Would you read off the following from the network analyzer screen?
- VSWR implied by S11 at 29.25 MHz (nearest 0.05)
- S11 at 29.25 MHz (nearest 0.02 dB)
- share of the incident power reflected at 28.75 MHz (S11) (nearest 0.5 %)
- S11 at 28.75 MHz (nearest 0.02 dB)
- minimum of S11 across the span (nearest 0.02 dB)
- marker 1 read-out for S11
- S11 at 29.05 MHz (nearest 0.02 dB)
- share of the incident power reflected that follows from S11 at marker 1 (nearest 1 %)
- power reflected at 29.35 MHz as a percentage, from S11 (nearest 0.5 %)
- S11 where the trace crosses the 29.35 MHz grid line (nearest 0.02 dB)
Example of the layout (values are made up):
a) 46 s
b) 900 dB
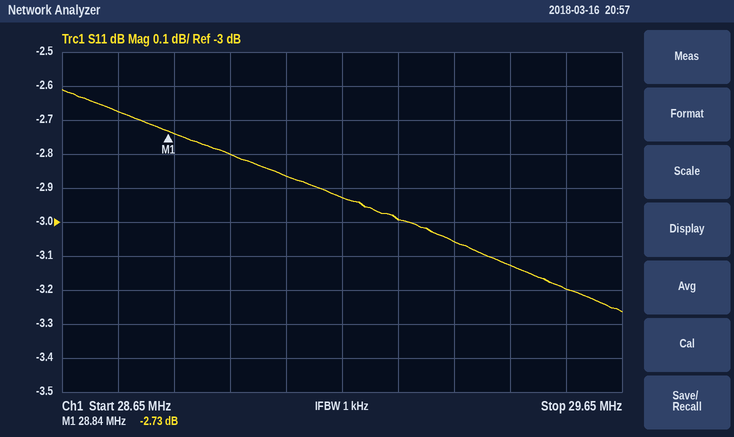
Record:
a) 5.85
b) -3.00 dB
c) 54.0 %
d) -2.68 dB
e) -3.26 dB
f) -2.73 dB
g) -2.86 dB
h) 53 %
i) 49.5 %
j) -3.06 dB
